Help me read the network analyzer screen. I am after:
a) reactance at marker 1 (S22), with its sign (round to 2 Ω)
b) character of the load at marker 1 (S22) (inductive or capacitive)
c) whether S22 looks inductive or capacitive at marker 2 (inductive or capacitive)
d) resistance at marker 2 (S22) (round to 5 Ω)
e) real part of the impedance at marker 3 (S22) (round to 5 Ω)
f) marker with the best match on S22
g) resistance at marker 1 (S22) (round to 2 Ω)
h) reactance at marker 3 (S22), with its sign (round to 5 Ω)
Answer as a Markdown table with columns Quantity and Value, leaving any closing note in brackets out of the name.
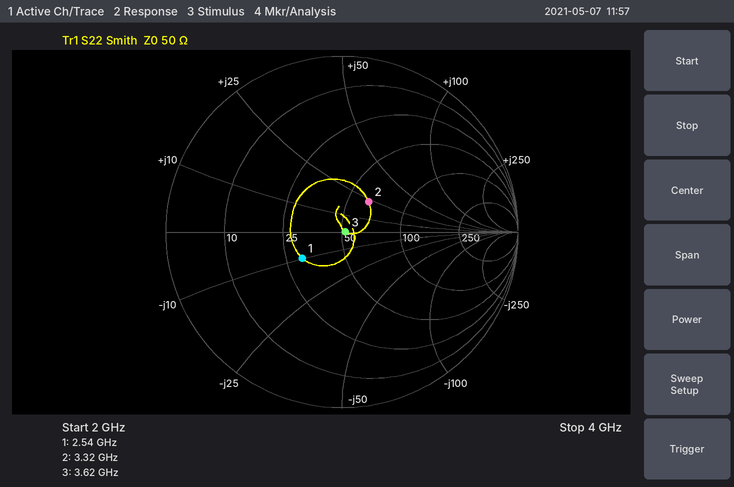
| Quantity | Value |
|---|---|
| reactance at marker 1 (S22), with its sign | -10 Ω |
| character of the load at marker 1 (S22) | capacitive |
| whether S22 looks inductive or capacitive at marker 2 | inductive |
| resistance at marker 2 (S22) | 65 Ω |
| real part of the impedance at marker 3 (S22) | 50 Ω |
| marker with the best match on S22 | marker 3 |
| resistance at marker 1 (S22) | 30 Ω |
| reactance at marker 3 (S22), with its sign | 0 Ω |
